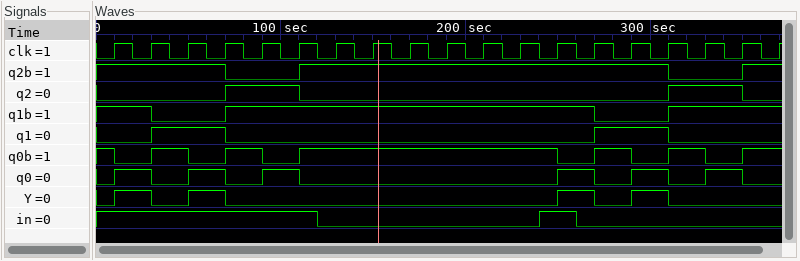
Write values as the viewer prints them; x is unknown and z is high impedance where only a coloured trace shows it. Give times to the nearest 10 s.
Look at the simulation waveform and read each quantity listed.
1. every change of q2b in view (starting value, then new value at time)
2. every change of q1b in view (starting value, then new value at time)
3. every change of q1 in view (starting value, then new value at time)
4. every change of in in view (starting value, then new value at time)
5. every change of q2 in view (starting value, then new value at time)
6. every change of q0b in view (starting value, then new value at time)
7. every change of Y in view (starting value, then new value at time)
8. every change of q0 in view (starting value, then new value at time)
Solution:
1, 0 at 70 s, 1 at 110 s, 0 at 310 s, 1 at 350 s
1, 0 at 30 s, 1 at 70 s, 0 at 270 s, 1 at 310 s
0, 1 at 30 s, 0 at 70 s, 1 at 270 s, 0 at 310 s
1, 0 at 120 s, 1 at 240 s, 0 at 260 s
0, 1 at 70 s, 0 at 110 s, 1 at 310 s, 0 at 350 s
1, 0 at 10 s, 1 at 30 s, 0 at 50 s, 1 at 70 s, 0 at 90 s, 1 at 110 s, 0 at 250 s, 1 at 270 s, 0 at 290 s, 1 at 310 s, 0 at 330 s, 1 at 350 s
0, 1 at 10 s, 0 at 30 s, 1 at 50 s, 0 at 70 s, 1 at 250 s, 0 at 270 s, 1 at 290 s, 0 at 310 s
0, 1 at 10 s, 0 at 30 s, 1 at 50 s, 0 at 70 s, 1 at 90 s, 0 at 110 s, 1 at 250 s, 0 at 270 s, 1 at 290 s, 0 at 310 s, 1 at 330 s, 0 at 350 s
